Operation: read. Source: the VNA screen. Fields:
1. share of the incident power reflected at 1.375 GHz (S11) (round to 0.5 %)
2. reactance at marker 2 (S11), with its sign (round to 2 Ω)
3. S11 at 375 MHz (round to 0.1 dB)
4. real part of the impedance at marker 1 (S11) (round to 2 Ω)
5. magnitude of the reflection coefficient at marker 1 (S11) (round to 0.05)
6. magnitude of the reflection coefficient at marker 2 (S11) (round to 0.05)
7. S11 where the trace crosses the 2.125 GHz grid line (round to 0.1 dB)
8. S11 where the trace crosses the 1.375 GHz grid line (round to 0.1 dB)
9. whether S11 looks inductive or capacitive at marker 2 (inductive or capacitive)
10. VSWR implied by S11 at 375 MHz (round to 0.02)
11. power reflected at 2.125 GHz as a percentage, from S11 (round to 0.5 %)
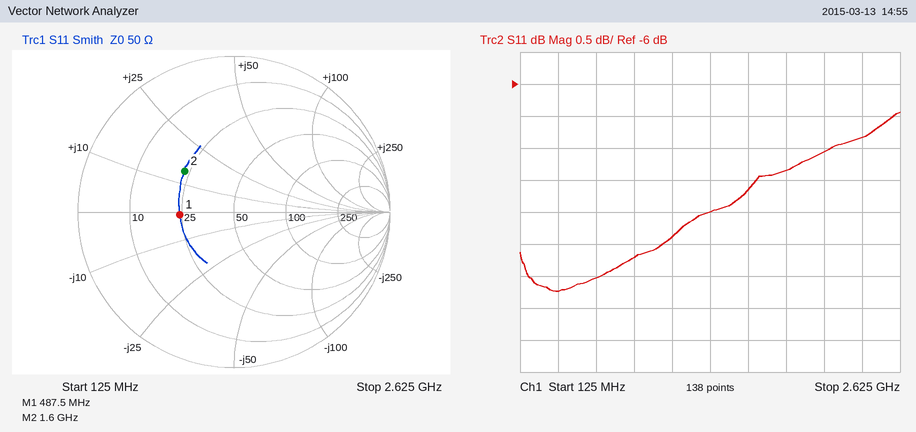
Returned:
16.0 %
+14 Ω
-9.2 dB
24 Ω
0.35
0.40
-7.1 dB
-8.0 dB
inductive
2.06
19.5 %
